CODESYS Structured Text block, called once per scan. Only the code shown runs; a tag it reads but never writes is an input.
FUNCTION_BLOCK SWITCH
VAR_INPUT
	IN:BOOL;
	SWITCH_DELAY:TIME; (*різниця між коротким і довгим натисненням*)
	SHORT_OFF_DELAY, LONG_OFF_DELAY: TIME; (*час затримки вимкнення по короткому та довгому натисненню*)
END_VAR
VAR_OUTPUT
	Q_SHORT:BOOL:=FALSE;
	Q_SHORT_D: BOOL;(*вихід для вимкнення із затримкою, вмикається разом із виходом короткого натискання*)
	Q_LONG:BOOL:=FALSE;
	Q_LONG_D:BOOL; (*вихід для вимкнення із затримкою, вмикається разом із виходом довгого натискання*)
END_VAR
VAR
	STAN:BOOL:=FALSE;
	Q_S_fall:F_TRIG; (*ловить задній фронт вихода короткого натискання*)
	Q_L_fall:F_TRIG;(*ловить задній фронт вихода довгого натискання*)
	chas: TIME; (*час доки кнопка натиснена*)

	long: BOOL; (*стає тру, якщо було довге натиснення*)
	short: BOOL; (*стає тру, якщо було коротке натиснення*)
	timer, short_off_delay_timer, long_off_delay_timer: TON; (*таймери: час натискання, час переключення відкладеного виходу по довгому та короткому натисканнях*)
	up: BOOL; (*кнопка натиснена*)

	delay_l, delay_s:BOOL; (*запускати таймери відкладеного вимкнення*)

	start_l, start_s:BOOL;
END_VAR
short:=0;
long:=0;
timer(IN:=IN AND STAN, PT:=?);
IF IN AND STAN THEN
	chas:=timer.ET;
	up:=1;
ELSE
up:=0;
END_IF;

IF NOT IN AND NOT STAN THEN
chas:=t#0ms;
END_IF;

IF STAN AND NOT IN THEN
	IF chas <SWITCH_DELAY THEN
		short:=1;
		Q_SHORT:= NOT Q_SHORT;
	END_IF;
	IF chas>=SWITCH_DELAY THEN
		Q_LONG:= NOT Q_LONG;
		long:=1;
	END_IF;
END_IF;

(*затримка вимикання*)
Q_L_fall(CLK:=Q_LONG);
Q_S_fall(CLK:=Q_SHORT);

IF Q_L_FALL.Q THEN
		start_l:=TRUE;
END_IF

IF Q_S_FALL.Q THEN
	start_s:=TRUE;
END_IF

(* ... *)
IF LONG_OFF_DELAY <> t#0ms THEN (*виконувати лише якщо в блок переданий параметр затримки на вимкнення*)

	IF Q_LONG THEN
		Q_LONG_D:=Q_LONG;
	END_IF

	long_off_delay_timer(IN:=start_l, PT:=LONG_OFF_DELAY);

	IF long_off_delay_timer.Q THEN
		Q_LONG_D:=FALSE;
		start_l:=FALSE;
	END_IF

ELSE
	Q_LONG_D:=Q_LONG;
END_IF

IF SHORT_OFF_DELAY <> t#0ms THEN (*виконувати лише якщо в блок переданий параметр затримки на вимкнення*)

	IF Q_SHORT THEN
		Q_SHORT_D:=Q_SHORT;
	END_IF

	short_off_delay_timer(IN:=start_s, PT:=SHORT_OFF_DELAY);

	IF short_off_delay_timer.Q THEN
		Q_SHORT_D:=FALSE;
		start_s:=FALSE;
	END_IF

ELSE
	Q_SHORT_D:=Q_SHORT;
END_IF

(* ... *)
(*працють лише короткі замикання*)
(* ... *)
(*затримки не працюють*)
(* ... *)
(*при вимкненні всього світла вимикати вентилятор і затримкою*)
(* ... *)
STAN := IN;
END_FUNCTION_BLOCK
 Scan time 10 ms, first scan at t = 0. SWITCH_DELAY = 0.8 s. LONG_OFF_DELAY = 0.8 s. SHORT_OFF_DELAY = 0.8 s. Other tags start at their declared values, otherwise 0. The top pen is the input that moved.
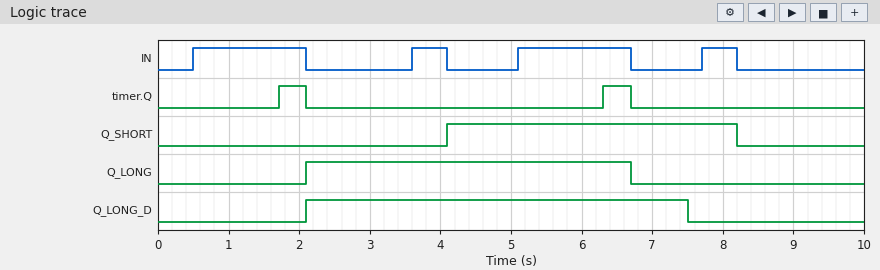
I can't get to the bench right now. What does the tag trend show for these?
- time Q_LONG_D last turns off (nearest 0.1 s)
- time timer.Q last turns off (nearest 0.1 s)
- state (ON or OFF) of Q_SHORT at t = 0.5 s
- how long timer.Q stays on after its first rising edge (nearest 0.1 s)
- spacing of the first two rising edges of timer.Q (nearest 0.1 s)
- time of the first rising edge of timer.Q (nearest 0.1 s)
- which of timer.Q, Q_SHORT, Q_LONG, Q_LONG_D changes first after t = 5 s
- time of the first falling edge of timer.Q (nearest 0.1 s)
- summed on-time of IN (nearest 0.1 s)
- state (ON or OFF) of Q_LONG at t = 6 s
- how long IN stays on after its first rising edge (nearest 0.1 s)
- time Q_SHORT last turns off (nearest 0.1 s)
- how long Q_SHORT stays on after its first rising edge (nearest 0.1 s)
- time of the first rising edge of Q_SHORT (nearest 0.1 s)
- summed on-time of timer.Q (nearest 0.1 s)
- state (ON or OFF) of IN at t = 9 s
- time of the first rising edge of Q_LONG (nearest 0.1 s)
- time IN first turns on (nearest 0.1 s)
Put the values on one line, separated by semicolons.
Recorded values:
7.5 s; 6.7 s; OFF; 0.4 s; 4.6 s; 1.7 s; timer.Q; 2.1 s; 4.2 s; ON; 1.6 s; 8.2 s; 4.1 s; 4.1 s; 0.8 s; OFF; 2.1 s; 0.5 s
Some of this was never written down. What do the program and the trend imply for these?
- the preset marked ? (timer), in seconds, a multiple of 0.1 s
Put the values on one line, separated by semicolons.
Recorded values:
1.2 s
